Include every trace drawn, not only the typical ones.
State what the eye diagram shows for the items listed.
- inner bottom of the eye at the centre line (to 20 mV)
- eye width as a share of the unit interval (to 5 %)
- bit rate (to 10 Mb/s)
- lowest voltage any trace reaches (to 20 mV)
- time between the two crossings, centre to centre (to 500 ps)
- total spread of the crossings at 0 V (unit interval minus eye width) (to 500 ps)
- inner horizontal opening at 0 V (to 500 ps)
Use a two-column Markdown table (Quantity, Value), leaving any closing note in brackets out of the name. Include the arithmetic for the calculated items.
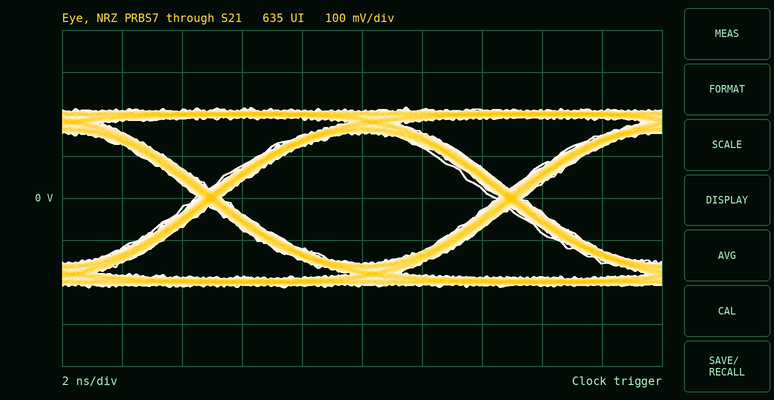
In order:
| Quantity | Value |
|---|---|
| inner bottom of the eye at the centre line | -160 mV |
| eye width as a share of the unit interval | 9.0 ns / 10.0 ns ≈ 90 % |
| bit rate | 100 Mb/s |
| lowest voltage any trace reaches | -220 mV |
| time between the two crossings, centre to centre | 10.0 ns |
| total spread of the crossings at 0 V (unit interval minus eye width) | 1.0 ns |
| inner horizontal opening at 0 V | 9.0 ns |
